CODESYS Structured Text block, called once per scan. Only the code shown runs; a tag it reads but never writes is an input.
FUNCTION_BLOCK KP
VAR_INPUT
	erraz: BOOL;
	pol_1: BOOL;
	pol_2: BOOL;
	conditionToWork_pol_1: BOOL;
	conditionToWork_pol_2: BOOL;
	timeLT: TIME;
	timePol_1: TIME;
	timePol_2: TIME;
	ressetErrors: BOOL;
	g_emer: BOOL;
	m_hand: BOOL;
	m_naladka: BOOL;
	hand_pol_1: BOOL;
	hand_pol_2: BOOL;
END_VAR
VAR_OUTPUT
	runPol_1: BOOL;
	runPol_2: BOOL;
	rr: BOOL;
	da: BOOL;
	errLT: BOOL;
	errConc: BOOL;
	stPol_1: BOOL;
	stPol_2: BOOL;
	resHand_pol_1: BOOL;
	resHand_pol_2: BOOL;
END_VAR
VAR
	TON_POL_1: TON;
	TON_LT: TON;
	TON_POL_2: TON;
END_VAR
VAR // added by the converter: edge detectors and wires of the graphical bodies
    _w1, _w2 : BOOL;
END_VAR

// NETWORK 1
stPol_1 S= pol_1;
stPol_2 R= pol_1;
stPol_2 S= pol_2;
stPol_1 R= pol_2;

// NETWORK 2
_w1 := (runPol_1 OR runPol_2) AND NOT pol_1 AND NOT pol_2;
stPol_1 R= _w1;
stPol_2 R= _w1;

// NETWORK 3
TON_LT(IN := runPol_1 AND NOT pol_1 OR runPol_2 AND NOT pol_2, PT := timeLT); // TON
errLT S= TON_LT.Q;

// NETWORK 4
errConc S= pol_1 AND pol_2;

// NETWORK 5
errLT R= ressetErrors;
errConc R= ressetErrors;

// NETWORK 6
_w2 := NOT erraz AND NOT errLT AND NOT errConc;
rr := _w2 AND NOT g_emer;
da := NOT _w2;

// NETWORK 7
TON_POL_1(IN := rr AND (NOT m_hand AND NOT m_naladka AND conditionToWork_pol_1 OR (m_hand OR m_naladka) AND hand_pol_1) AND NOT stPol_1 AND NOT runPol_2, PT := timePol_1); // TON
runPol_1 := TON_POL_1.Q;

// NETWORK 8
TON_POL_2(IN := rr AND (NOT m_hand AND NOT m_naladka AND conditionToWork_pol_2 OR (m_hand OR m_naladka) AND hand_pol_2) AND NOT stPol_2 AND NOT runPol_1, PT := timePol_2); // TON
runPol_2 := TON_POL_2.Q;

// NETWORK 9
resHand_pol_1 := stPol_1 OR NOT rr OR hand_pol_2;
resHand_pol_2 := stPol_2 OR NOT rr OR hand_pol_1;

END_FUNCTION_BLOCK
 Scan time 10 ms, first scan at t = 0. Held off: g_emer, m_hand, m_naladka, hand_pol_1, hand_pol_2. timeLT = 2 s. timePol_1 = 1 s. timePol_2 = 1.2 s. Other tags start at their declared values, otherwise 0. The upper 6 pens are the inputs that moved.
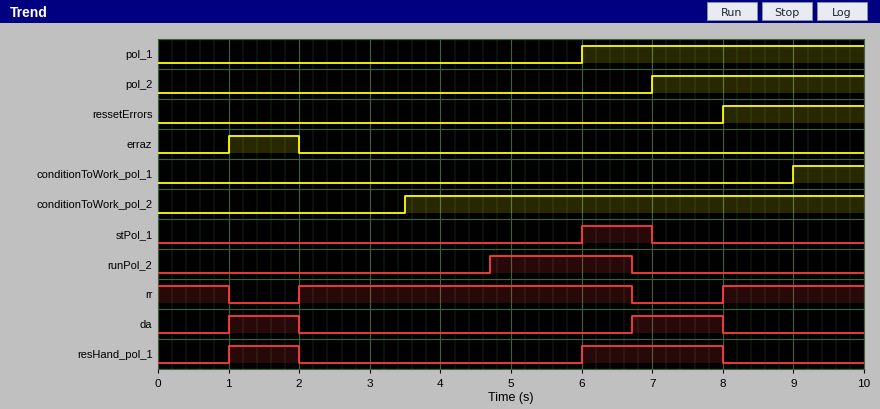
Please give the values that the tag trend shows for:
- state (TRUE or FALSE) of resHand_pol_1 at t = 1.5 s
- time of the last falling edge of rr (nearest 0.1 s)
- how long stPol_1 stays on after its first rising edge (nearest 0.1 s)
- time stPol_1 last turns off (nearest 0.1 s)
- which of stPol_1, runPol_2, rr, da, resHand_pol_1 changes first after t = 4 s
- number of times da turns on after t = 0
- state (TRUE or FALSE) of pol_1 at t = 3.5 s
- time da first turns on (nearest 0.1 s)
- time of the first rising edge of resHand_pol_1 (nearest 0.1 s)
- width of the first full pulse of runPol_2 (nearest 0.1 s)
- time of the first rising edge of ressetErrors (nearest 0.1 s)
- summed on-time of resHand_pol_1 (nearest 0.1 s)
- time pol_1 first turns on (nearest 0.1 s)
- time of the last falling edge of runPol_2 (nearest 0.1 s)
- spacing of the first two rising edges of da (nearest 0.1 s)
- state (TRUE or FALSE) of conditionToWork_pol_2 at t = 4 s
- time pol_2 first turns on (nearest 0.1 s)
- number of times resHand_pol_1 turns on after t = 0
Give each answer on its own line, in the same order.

TRUE
6.7 s
1.0 s
7.0 s
runPol_2
2
FALSE
1.0 s
1.0 s
2.0 s
8.0 s
3.0 s
6.0 s
6.7 s
5.7 s
TRUE
7.0 s
2
